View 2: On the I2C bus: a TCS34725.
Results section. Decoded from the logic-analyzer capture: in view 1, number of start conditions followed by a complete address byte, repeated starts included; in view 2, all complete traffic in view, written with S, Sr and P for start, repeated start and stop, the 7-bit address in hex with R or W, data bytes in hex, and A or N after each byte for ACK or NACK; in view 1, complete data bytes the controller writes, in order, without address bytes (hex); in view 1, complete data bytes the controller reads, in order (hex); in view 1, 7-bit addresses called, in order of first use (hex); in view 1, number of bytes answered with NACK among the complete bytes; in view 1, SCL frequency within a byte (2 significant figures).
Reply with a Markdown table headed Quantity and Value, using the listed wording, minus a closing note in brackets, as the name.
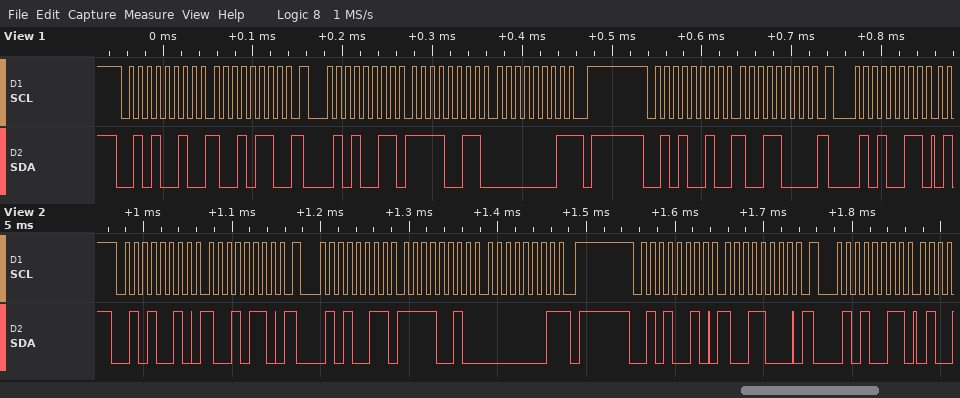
| Quantity | Value |
|---|---|
| in view 1, number of start conditions followed by a complete address byte, repeated starts included | 4 |
| in view 2, all complete traffic in view, written with S, Sr and P for start, repeated start and stop, the 7-bit address in hex with R or W, data bytes in hex, and A or N after each byte for ACK or NACK | S 29W A 96 A Sr 29R A F2 A 01 N P S 29W A 98 A Sr 29R A |
| in view 1, complete data bytes the controller writes, in order, without address bytes | 96 98 |
| in view 1, complete data bytes the controller reads, in order | F3 01 |
| in view 1, 7-bit addresses called, in order of first use | 0x29 |
| in view 1, number of bytes answered with NACK among the complete bytes | 1 |
| in view 1, SCL frequency within a byte | 100 kHz |
